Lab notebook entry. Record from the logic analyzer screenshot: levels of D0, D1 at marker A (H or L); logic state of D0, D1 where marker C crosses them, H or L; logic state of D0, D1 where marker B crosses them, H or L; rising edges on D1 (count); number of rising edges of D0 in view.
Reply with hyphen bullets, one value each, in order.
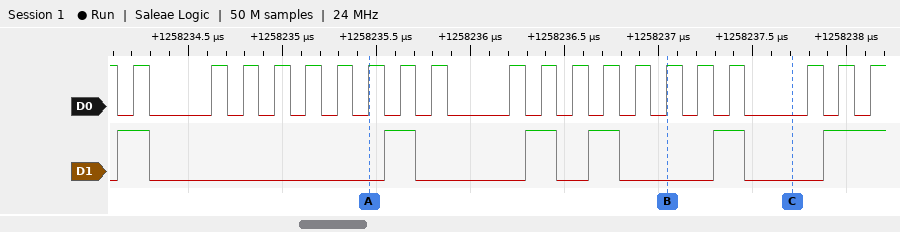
- D0=H, D1=L
- D0=L, D1=L
- D0=H, D1=L
- 6
- 20
